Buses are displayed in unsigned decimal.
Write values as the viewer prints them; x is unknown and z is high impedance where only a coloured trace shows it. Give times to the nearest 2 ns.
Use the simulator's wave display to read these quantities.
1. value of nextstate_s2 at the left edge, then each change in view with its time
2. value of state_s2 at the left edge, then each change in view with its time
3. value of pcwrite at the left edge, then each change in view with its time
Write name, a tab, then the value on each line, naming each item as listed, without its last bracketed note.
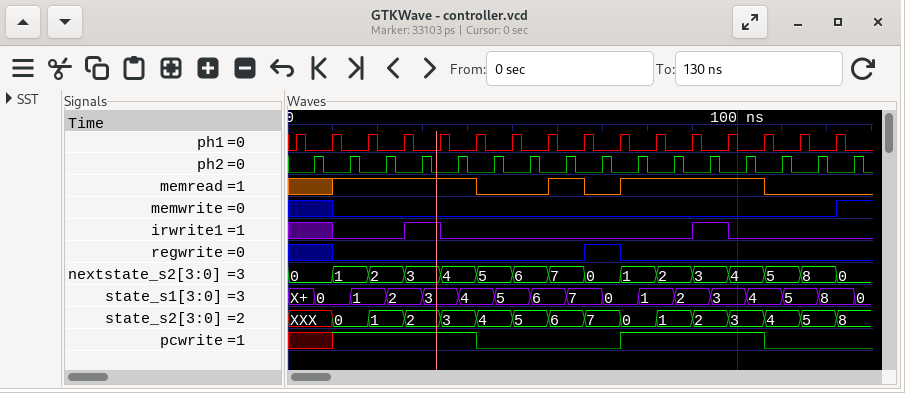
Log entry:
value of nextstate_s2 at the left edge, then each change in view with its time	0, 1 at 10 ns, 2 at 18 ns, 3 at 26 ns, 4 at 34 ns, 5 at 42 ns, 6 at 50 ns, 7 at 58 ns, 0 at 66 ns, 1 at 74 ns, 2 at 82 ns, 3 at 90 ns, 4 at 98 ns, 5 at 106 ns, 8 at 114 ns, 0 at 122 ns
value of state_s2 at the left edge, then each change in view with its time	XXX, 0 at 10 ns, 1 at 18 ns, 2 at 26 ns, 3 at 34 ns, 4 at 42 ns, 5 at 50 ns, 6 at 58 ns, 7 at 66 ns, 0 at 74 ns, 1 at 82 ns, 2 at 90 ns, 3 at 98 ns, 4 at 106 ns, 5 at 114 ns, 8 at 122 ns
value of pcwrite at the left edge, then each change in view with its time	x, 1 at 10 ns, 0 at 42 ns, 1 at 74 ns, 0 at 106 ns
